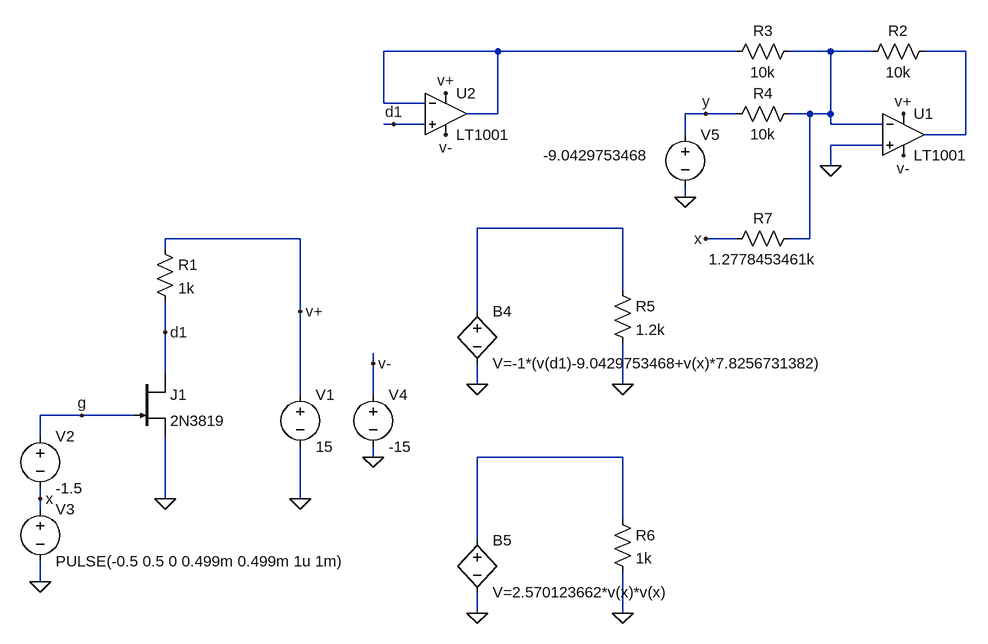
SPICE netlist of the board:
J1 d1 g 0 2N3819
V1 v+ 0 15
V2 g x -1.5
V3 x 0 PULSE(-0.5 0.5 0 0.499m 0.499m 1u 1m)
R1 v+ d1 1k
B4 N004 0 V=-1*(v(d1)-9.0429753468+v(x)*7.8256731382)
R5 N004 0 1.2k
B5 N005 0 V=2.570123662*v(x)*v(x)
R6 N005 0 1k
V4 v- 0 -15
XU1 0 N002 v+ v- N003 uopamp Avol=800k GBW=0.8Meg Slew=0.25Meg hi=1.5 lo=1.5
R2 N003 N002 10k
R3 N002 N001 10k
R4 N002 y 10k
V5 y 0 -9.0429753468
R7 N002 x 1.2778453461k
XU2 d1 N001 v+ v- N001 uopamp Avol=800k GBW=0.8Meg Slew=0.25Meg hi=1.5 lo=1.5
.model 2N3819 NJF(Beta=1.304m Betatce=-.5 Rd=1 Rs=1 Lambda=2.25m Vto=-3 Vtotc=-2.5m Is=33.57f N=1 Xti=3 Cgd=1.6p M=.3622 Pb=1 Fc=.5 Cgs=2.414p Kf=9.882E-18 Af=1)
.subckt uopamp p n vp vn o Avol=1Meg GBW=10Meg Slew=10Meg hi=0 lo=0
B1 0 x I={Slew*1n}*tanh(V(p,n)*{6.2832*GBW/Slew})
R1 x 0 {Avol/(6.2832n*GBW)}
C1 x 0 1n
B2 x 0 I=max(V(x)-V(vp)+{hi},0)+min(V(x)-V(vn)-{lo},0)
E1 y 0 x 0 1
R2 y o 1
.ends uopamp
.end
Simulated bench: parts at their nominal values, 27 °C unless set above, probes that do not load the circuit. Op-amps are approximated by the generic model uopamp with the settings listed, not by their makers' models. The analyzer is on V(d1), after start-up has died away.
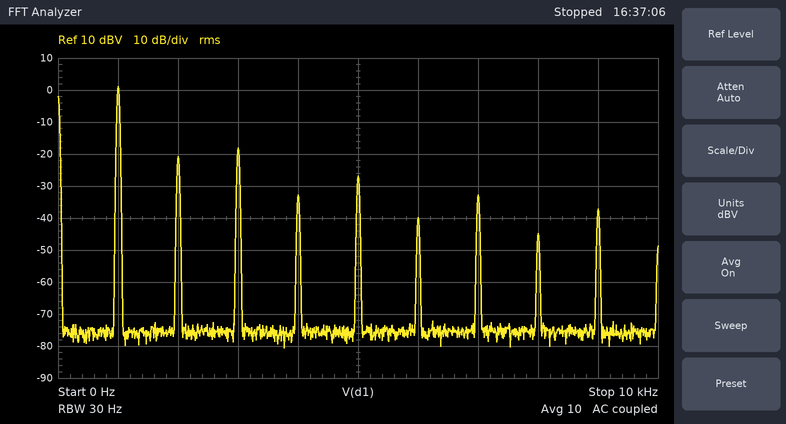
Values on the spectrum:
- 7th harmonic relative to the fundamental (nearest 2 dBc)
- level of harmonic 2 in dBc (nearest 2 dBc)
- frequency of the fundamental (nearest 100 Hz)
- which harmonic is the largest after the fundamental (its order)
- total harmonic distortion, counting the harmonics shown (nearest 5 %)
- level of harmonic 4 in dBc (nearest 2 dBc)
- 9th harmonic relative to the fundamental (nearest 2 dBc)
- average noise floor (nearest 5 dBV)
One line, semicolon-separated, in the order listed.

-34 dBc; -22 dBc; 1.0 kHz; 3; 15 %; -34 dBc; -38 dBc; -75 dBV
